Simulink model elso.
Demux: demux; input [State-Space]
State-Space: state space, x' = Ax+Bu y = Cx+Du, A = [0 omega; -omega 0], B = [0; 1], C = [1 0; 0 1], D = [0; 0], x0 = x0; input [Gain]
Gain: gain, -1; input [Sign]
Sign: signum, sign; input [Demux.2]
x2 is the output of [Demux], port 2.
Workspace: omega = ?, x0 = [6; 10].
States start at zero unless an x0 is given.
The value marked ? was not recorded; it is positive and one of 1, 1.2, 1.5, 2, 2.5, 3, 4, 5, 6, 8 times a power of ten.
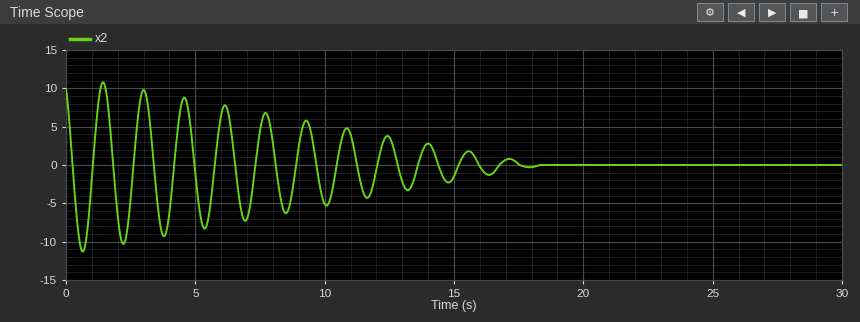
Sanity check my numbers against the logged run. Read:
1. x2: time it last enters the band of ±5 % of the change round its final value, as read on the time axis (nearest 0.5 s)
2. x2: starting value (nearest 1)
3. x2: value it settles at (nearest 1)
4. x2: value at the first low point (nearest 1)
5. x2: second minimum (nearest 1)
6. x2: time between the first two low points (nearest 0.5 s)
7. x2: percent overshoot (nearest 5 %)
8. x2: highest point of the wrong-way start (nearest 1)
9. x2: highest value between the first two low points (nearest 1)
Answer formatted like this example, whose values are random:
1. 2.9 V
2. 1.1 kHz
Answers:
1. 17.5 s
2. 10
3. 0
4. -11
5. -10
6. 1.5 s
7. 115 %
8. 11
9. 11
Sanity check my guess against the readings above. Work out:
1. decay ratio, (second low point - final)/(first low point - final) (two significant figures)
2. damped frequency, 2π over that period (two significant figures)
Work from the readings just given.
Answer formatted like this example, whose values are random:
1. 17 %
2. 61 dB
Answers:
1. 0.91
2. 4.2 rad/s
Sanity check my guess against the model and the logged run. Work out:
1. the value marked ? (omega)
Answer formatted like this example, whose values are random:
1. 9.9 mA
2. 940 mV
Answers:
1. 4
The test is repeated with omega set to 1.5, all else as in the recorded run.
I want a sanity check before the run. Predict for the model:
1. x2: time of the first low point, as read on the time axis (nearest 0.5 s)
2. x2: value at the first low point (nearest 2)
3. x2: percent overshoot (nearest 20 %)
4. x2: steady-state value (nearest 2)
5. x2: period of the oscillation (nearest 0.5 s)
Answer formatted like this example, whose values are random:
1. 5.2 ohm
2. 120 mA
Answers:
1. 1.5 s
2. -10
3. 100 %
4. 0
5. 4.0 s
